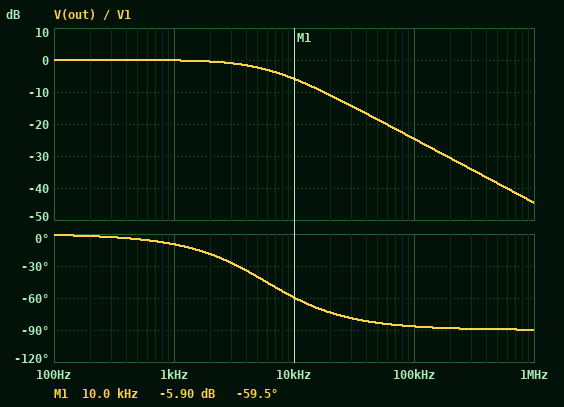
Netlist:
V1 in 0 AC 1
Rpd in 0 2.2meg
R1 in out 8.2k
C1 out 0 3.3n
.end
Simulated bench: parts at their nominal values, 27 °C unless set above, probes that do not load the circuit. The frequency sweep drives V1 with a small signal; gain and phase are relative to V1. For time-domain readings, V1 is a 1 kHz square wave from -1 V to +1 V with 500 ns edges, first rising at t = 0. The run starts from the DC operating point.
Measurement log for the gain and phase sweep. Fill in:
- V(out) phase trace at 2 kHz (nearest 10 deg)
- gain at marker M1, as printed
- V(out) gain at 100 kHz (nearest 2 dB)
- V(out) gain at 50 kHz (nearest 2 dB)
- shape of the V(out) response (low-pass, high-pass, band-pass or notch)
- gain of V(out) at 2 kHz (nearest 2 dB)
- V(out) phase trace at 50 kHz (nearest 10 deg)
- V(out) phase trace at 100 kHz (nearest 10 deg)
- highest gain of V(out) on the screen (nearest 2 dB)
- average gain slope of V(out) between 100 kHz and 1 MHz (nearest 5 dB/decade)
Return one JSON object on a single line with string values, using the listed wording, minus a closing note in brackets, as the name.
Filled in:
{"V(out) phase trace at 2 kHz": "-20 deg", "gain at marker M1, as printed": "-5.90 dB", "V(out) gain at 100 kHz": "-24 dB", "V(out) gain at 50 kHz": "-18 dB", "shape of the V(out) response": "low-pass", "gain of V(out) at 2 kHz": "0 dB", "V(out) phase trace at 50 kHz": "-80 deg", "V(out) phase trace at 100 kHz": "-90 deg", "highest gain of V(out) on the screen": "0 dB", "average gain slope of V(out) between 100 kHz and 1 MHz": "-20 dB/decade"}
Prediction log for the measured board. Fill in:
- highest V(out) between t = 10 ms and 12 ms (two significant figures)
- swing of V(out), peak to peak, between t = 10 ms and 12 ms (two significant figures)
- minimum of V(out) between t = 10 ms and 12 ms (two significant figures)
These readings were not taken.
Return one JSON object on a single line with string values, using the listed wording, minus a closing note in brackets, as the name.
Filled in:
{"highest V(out) between t = 10 ms and 12 ms": "1.0 V", "swing of V(out), peak to peak, between t = 10 ms and 12 ms": "2.0 V", "minimum of V(out) between t = 10 ms and 12 ms": "-1.0 V"}
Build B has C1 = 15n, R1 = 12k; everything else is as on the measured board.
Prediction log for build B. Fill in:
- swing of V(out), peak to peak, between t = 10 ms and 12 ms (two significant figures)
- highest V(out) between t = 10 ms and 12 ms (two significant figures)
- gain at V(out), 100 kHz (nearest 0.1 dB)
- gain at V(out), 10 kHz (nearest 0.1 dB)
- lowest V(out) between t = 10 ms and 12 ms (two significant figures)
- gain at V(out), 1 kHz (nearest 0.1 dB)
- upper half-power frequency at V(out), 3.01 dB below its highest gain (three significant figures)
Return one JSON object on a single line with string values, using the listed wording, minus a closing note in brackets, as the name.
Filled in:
{"swing of V(out), peak to peak, between t = 10 ms and 12 ms": "1.8 V", "highest V(out) between t = 10 ms and 12 ms": "880 mV", "gain at V(out), 100 kHz": "-41.1 dB", "gain at V(out), 10 kHz": "-21.1 dB", "lowest V(out) between t = 10 ms and 12 ms": "-880 mV", "gain at V(out), 1 kHz": "-3.6 dB", "upper half-power frequency at V(out), 3.01 dB below its highest gain": "884 Hz"}
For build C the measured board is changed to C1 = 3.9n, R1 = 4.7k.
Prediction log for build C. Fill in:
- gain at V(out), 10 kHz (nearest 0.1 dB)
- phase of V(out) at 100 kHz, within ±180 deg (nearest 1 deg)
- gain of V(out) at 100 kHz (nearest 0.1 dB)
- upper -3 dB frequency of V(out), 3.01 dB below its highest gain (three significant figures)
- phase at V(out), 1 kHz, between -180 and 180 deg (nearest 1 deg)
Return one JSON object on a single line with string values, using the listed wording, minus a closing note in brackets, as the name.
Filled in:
{"gain at V(out), 10 kHz": "-3.7 dB", "phase of V(out) at 100 kHz, within ±180 deg": "-85 deg", "gain of V(out) at 100 kHz": "-21.3 dB", "upper -3 dB frequency of V(out), 3.01 dB below its highest gain": "8.68 kHz", "phase at V(out), 1 kHz, between -180 and 180 deg": "-7 deg"}
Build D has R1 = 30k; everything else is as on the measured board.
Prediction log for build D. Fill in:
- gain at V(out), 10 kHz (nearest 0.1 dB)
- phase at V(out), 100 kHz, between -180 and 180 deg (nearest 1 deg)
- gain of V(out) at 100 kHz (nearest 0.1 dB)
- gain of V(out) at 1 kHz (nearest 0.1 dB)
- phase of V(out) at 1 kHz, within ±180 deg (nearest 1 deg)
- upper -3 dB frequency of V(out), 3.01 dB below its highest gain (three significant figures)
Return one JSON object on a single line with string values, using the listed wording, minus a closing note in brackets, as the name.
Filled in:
{"gain at V(out), 10 kHz": "-16.0 dB", "phase at V(out), 100 kHz, between -180 and 180 deg": "-89 deg", "gain of V(out) at 100 kHz": "-35.9 dB", "gain of V(out) at 1 kHz": "-1.4 dB", "phase of V(out) at 1 kHz, within ±180 deg": "-32 deg", "upper -3 dB frequency of V(out), 3.01 dB below its highest gain": "1.61 kHz"}
